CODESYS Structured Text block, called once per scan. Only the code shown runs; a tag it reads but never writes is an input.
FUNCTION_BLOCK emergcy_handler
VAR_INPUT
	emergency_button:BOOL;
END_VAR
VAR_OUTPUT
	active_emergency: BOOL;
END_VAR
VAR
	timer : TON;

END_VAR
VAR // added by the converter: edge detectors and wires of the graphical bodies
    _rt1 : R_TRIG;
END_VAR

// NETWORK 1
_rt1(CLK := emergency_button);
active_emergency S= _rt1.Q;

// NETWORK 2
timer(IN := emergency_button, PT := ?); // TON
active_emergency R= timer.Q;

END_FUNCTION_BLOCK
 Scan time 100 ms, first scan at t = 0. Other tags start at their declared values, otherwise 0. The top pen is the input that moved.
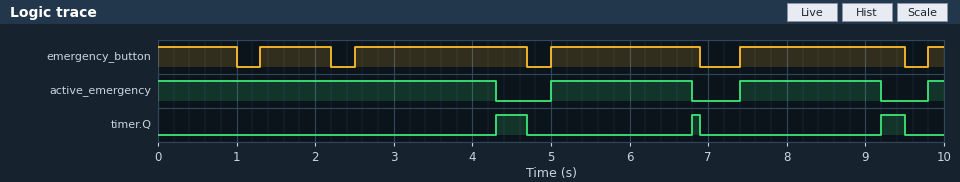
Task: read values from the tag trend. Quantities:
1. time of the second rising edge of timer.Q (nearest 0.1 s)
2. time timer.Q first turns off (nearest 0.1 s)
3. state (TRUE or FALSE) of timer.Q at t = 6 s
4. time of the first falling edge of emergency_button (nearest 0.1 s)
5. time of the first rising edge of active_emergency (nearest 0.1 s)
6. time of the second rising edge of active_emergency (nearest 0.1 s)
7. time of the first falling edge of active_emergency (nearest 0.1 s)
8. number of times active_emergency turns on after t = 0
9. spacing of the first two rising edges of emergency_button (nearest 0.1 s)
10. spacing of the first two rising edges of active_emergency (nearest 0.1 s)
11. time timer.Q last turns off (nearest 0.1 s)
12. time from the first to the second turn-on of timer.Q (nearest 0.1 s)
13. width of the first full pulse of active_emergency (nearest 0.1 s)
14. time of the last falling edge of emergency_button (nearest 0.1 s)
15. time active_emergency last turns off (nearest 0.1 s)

6.8 s
4.7 s
FALSE
1.0 s
5.0 s
7.4 s
4.3 s
3
1.2 s
2.4 s
9.5 s
2.5 s
1.8 s
9.5 s
9.2 s
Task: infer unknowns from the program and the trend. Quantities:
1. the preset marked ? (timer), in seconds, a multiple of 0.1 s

1.8 s
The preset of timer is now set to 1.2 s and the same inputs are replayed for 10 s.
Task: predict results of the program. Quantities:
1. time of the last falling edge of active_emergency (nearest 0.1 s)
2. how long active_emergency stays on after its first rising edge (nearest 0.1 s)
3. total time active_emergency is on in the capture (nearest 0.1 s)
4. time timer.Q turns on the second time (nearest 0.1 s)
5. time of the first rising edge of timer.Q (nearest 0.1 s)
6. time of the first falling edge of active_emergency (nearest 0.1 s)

8.6 s
1.2 s
6.3 s
6.2 s
3.7 s
3.7 s
